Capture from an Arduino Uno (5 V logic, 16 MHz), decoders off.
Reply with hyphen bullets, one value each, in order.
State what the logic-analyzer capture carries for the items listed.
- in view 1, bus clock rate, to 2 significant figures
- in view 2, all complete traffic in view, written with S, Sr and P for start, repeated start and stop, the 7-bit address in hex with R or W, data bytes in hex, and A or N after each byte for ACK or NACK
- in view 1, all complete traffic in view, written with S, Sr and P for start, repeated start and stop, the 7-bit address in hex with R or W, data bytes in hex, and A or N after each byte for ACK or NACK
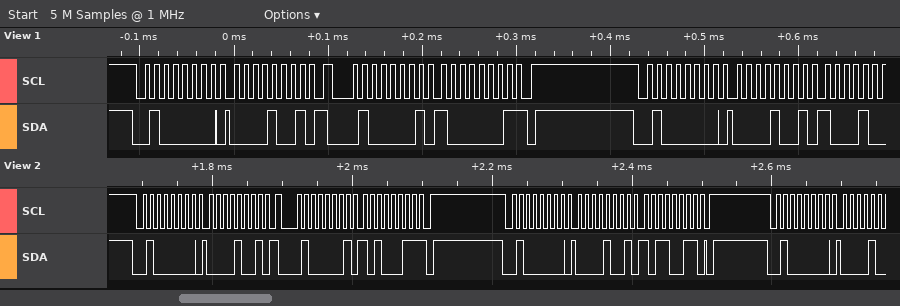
- 100 kHz
- S 20W A 09 A Sr 20R A A3 N P S 20W A 09 A B3 A P S 20W A
- S 20W A 09 A Sr 20R A 81 N P S 20W A 09 A
